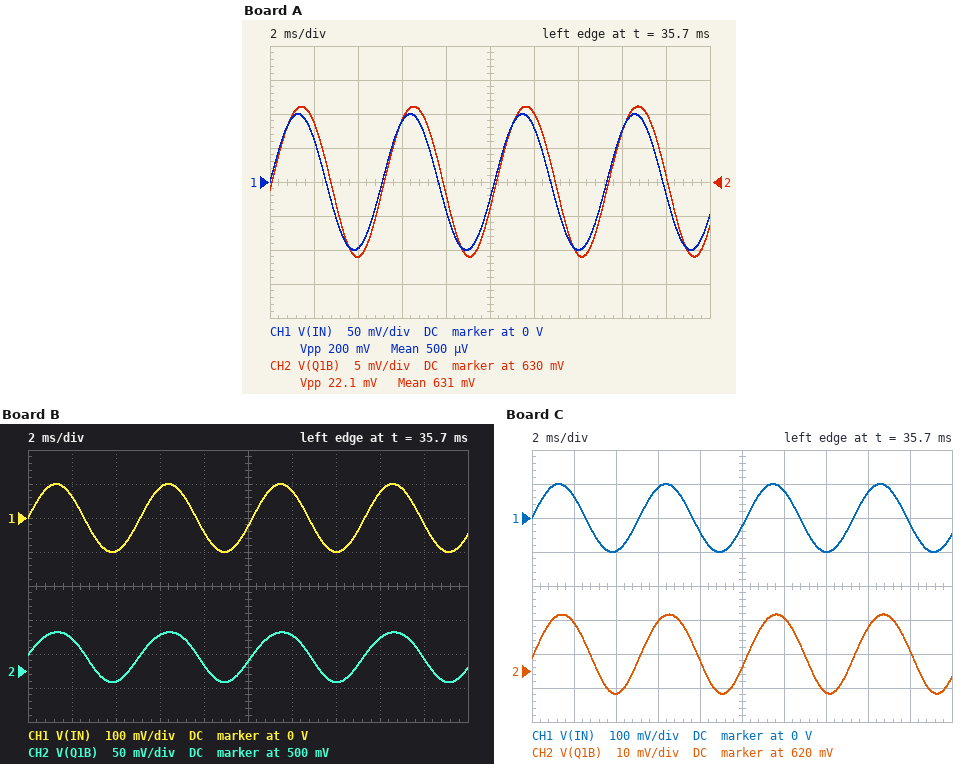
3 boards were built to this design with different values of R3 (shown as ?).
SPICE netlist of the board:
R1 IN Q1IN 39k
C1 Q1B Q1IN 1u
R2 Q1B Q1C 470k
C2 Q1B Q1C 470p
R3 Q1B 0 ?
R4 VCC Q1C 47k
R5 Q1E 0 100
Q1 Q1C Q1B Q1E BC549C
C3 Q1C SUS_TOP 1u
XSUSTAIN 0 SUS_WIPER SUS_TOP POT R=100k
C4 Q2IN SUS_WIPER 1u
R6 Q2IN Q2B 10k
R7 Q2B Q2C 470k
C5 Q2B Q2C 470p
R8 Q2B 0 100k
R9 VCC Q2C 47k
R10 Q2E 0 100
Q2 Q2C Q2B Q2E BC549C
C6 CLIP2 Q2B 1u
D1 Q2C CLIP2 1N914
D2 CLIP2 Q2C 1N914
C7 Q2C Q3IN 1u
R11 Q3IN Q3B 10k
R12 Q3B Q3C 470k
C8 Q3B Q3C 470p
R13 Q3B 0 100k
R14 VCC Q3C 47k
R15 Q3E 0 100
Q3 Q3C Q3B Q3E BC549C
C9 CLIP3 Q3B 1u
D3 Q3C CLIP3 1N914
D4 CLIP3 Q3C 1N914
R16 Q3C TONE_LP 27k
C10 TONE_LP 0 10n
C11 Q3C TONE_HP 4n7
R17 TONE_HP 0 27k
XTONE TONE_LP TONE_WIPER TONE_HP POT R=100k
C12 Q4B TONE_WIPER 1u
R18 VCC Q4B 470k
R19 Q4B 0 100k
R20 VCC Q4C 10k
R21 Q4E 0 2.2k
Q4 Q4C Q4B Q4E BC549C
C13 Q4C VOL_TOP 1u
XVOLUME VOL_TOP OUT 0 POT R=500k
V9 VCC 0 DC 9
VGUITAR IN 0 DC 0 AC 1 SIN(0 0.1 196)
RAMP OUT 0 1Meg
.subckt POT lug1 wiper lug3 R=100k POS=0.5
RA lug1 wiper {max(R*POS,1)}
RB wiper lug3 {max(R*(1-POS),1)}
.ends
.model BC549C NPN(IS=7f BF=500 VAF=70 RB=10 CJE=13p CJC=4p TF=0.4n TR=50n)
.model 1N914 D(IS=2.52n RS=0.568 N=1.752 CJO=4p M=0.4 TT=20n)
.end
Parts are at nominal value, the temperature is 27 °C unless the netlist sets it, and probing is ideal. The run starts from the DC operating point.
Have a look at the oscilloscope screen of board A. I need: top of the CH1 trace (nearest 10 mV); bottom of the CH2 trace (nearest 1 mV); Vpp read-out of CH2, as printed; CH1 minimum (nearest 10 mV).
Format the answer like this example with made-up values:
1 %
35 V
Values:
100 mV
619 mV
22.1 mV
-100 mV
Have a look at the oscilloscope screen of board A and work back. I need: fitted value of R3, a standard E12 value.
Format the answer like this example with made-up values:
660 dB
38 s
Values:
330 kΩ
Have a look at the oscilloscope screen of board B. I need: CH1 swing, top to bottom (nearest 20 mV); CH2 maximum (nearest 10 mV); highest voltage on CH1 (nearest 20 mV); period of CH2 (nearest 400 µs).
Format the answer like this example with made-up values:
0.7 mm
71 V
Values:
200 mV
560 mV
100 mV
5.2 ms
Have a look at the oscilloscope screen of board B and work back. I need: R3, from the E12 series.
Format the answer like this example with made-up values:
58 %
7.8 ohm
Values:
33 kΩ
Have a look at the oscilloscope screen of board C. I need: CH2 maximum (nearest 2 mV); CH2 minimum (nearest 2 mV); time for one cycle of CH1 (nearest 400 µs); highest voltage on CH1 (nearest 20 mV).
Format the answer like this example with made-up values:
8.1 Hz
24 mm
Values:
636 mV
614 mV
5.2 ms
100 mV
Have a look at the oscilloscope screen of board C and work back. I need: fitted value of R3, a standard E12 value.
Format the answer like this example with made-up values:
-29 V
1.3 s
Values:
180 kΩ
